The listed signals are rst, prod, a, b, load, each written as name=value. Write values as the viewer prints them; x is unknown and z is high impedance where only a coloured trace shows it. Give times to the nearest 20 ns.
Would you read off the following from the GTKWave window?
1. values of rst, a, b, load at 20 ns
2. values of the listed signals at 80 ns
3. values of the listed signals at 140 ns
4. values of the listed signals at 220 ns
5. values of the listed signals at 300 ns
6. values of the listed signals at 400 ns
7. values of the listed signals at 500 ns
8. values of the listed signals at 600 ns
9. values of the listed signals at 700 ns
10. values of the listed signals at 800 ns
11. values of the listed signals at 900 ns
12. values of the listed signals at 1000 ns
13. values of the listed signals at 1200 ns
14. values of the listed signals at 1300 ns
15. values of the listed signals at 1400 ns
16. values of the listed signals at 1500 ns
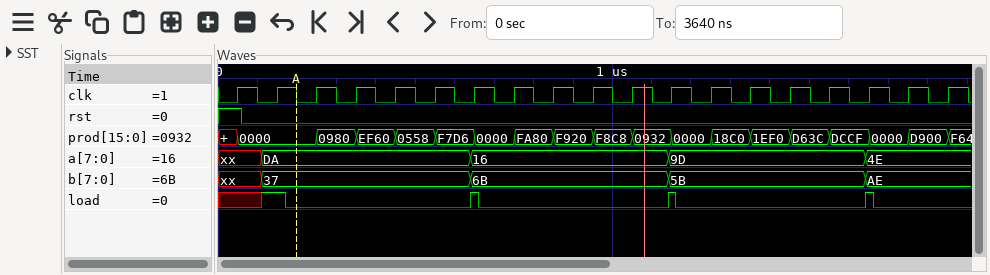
rst=1, a=xx, b=xx, load=x
rst=0, prod=0000, a=xx, b=xx, load=x
rst=0, prod=0000, a=DA, b=37, load=1
rst=0, prod=0000, a=DA, b=37, load=0
rst=0, prod=0980, a=DA, b=37, load=0
rst=0, prod=EF60, a=DA, b=37, load=0
rst=0, prod=0558, a=DA, b=37, load=0
rst=0, prod=F7D6, a=DA, b=37, load=0
rst=0, prod=0000, a=16, b=6B, load=0
rst=0, prod=FA80, a=16, b=6B, load=0
rst=0, prod=F920, a=16, b=6B, load=0
rst=0, prod=F8C8, a=16, b=6B, load=0
rst=0, prod=0000, a=9D, b=5B, load=0
rst=0, prod=18C0, a=9D, b=5B, load=0
rst=0, prod=1EF0, a=9D, b=5B, load=0
rst=0, prod=D63C, a=9D, b=5B, load=0
